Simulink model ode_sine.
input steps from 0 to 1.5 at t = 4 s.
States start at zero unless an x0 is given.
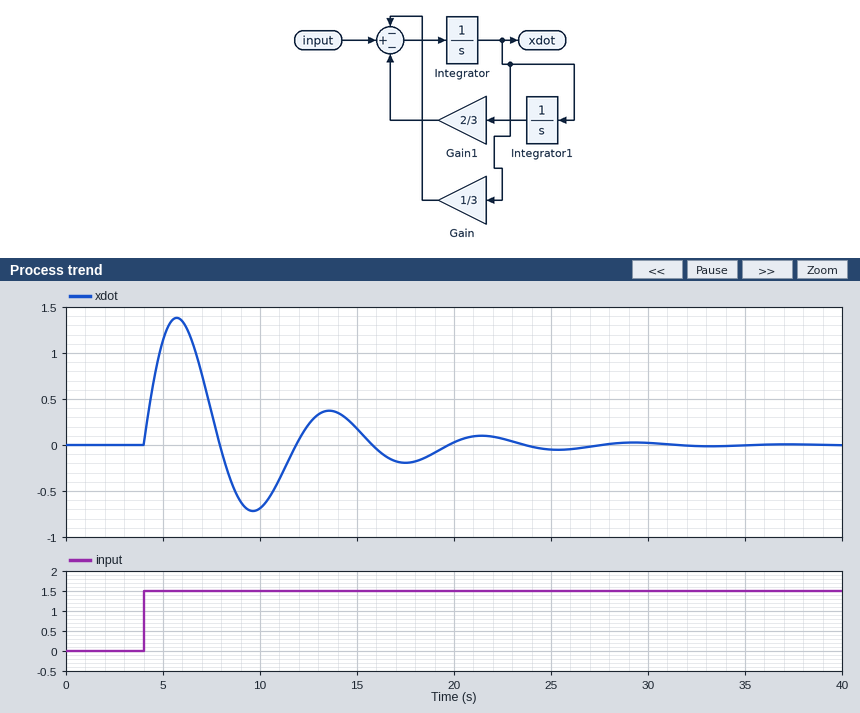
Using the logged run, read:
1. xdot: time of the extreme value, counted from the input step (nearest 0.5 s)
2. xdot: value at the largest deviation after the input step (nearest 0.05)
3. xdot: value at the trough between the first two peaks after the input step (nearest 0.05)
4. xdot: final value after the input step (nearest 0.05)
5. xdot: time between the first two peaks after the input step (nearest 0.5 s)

1.5 s
1.40
-0.70
0.00
8.0 s
